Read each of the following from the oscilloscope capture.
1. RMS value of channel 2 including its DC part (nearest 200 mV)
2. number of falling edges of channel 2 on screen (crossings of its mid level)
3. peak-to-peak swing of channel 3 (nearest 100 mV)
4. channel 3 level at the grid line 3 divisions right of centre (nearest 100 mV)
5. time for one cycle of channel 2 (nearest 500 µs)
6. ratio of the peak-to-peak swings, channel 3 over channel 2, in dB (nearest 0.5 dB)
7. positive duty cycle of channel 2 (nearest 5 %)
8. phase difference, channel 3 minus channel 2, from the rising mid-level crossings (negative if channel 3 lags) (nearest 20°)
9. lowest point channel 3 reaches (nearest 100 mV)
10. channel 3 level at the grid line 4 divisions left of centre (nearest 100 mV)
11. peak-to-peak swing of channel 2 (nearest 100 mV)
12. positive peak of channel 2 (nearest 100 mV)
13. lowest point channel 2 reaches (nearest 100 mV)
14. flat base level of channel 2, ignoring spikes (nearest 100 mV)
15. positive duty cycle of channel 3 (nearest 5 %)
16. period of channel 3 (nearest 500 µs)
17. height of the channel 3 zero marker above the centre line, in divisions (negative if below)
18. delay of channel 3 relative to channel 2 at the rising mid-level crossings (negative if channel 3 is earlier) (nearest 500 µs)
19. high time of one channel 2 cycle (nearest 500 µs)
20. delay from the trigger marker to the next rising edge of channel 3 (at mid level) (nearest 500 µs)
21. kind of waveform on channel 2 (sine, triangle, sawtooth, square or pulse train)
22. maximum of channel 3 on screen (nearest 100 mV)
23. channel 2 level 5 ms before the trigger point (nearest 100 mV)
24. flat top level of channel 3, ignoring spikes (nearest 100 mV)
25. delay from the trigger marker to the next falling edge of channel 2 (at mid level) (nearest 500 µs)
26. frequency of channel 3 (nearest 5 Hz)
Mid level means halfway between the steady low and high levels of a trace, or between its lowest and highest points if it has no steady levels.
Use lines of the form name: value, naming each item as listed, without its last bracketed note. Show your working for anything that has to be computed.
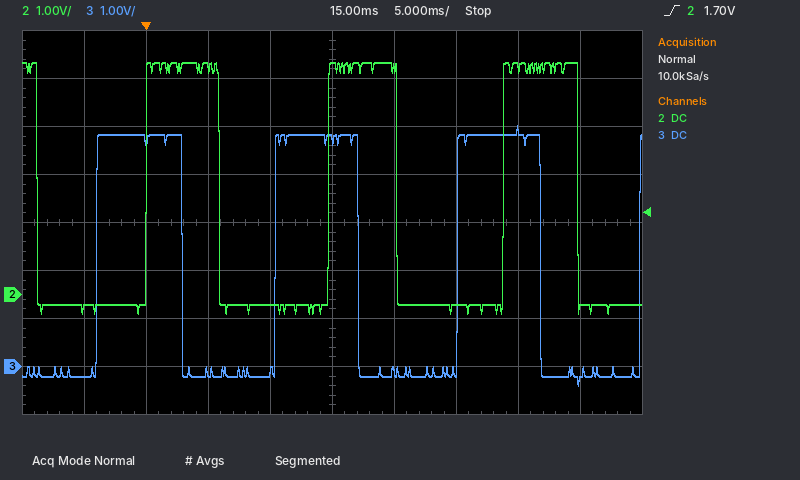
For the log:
RMS value of channel 2 including its DC part: √(0.4 × (4.8 V)² + 0.6 × (-200 mV)²) ≈ 3.0 V
number of falling edges of channel 2 on screen: 4
peak-to-peak swing of channel 3: 5.0 V − (-400 mV) = 5.4 V
channel 3 level at the grid line 3 divisions right of centre: 4.9 V
time for one cycle of channel 2: 14.5 ms
ratio of the peak-to-peak swings, channel 3 over channel 2, in dB: 20 log10(5.4 V / 5.2 V) ≈ 0.328 dB, so 0.5 dB to the nearest 0.5 dB
positive duty cycle of channel 2: 6.0 ms / 14.5 ms ≈ 41.4 %, so 40 % to the nearest 5 %
phase difference, channel 3 minus channel 2, from the rising mid-level crossings (negative if channel 3 lags): −360° × (-4.0 ms) / 14.5 ms ≈ +99.3°, so +100° to the nearest 20°
lowest point channel 3 reaches: -400 mV
channel 3 level at the grid line 4 divisions left of centre: -200 mV
peak-to-peak swing of channel 2: 4.8 V − (-400 mV) = 5.2 V
positive peak of channel 2: 4.8 V
lowest point channel 2 reaches: -400 mV
flat base level of channel 2, ignoring spikes: -200 mV
positive duty cycle of channel 3: 45 %
period of channel 3: 14.5 ms
height of the channel 3 zero marker above the centre line, in divisions: -3.0 div
delay of channel 3 relative to channel 2 at the rising mid-level crossings (negative if channel 3 is earlier): -4.0 ms
high time of one channel 2 cycle: 6.0 ms
delay from the trigger marker to the next rising edge of channel 3 (at mid level): 10.5 ms
kind of waveform on channel 2: pulse train
maximum of channel 3 on screen: 5.0 V
channel 2 level 5 ms before the trigger point: -300 mV
flat top level of channel 3, ignoring spikes: 4.8 V
delay from the trigger marker to the next falling edge of channel 2 (at mid level): 6.0 ms
frequency of channel 3: 1 / 14.5 ms ≈ 69.0 Hz, so 70 Hz to the nearest 5 Hz
